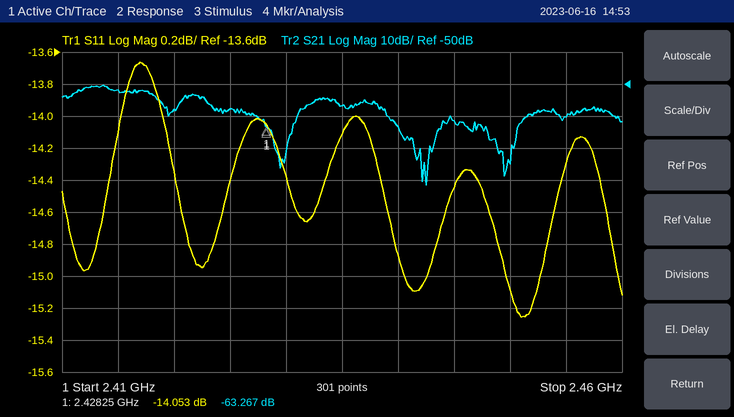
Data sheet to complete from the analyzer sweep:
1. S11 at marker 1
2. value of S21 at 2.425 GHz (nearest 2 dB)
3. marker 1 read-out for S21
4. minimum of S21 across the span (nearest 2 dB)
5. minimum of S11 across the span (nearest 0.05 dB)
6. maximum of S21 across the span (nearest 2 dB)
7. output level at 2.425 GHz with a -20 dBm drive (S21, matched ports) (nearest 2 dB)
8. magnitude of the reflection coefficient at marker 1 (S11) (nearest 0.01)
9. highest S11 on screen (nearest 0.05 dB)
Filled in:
-14.053 dB
-58 dB
-63.267 dB
-82 dB
-15.25 dB
-50 dB
-78 dBm
0.20
-13.65 dB
